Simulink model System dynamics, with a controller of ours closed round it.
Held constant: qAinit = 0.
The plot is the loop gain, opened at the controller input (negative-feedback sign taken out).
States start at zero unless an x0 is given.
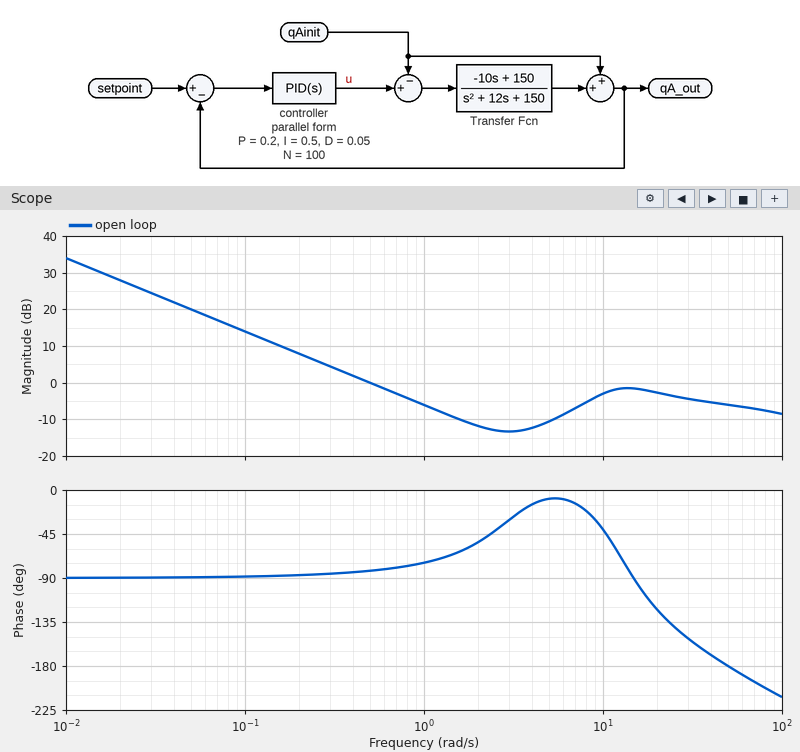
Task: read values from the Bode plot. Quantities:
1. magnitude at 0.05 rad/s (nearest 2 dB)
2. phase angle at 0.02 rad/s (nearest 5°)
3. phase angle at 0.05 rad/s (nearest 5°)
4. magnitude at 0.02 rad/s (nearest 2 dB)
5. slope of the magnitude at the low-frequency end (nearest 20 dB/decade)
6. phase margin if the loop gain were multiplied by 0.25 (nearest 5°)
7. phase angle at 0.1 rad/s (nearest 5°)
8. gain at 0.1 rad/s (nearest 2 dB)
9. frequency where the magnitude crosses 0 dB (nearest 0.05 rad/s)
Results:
20 dB
-90°
-90°
28 dB
-20 dB/decade
90°
-90°
14 dB
0.50 rad/s
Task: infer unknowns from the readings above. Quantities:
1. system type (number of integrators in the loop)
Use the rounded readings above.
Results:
1
